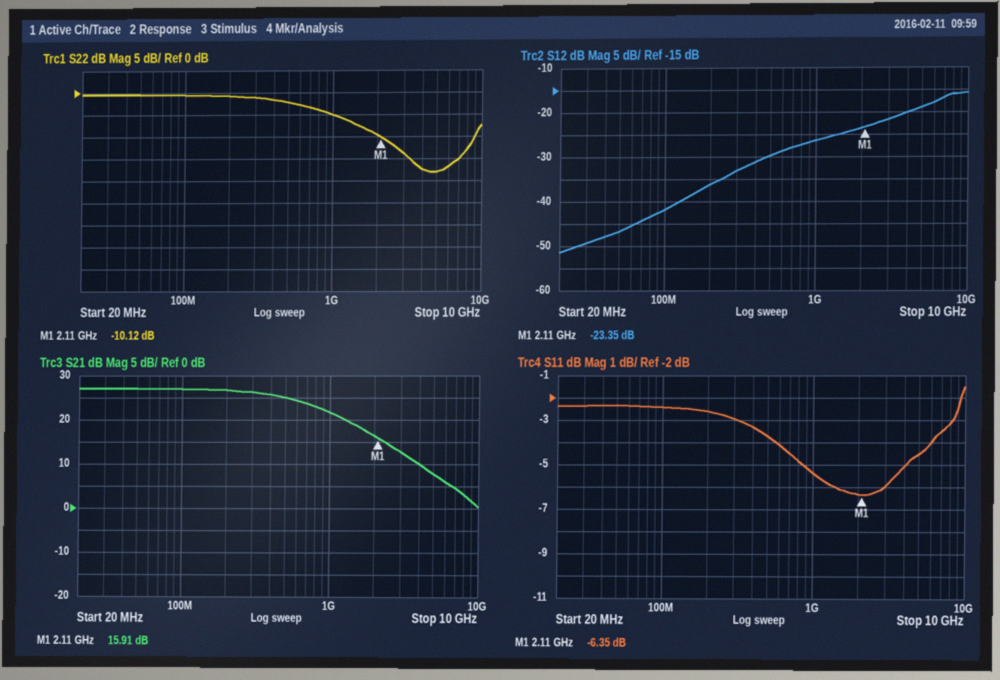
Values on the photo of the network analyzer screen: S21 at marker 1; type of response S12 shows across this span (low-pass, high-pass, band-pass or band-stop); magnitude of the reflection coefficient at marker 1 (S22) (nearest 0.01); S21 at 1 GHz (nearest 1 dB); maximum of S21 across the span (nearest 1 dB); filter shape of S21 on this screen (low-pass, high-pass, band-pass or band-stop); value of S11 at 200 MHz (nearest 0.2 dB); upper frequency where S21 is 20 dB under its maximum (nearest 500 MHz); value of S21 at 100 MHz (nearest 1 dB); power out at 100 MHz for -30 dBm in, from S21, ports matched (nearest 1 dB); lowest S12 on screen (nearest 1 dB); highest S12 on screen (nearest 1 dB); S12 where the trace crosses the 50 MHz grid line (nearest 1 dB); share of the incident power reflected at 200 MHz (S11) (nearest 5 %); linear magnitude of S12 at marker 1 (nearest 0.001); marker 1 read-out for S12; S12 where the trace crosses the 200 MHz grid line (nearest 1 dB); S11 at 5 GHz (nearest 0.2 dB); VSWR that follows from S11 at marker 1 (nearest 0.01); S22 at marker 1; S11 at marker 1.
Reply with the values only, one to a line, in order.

15.91 dB
high-pass
0.31
22 dB
27 dB
low-pass
-2.6 dB
5.5 GHz
27 dB
-3 dBm
-51 dB
-16 dB
-47 dB
55 %
0.068
-23.35 dB
-36 dB
-4.6 dB
2.86
-10.12 dB
-6.35 dB
